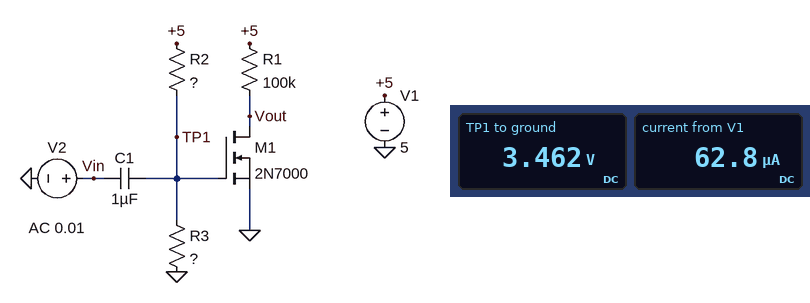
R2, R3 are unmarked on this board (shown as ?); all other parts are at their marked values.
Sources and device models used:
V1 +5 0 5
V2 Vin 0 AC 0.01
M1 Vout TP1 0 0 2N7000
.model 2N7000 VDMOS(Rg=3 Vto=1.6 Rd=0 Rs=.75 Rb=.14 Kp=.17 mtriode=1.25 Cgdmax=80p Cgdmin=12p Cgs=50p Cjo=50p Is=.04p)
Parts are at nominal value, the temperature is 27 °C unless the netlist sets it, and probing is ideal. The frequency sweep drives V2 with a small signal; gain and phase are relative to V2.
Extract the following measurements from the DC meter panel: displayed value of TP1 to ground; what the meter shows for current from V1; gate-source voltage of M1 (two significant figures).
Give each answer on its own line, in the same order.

3.462 V
62.8 µA
3.5 V
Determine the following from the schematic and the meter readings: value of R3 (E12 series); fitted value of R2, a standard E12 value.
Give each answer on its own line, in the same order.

270 kΩ
120 kΩ
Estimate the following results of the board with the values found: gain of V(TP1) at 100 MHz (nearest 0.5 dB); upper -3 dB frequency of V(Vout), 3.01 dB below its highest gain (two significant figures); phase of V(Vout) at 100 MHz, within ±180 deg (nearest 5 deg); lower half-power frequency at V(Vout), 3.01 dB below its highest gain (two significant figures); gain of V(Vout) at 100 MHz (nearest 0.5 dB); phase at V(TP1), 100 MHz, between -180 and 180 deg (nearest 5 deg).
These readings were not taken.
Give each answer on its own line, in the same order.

0 dB
1.6 GHz
60 deg
170 MHz
-15.5 dB
0 deg
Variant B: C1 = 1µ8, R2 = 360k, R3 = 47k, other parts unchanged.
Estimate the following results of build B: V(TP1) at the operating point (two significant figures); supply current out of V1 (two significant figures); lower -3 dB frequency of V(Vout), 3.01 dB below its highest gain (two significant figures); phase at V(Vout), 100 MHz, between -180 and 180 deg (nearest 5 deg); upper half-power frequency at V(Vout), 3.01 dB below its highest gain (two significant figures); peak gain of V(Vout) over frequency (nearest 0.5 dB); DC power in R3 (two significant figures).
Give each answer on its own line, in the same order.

580 mV
12 µA
44 kHz
-5 deg
780 MHz
-6.0 dB
7.1 µW
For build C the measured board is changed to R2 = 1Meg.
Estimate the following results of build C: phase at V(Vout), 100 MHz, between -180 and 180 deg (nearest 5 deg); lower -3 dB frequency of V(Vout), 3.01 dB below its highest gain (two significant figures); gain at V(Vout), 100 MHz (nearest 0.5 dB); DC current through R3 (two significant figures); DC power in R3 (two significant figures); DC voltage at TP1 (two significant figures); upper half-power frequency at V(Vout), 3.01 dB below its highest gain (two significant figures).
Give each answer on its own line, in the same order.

-5 deg
43 kHz
-6.0 dB
3.9 µA
4.2 µW
1.1 V
780 MHz
